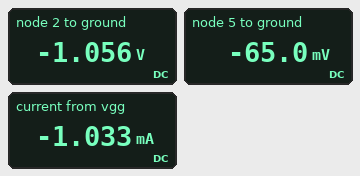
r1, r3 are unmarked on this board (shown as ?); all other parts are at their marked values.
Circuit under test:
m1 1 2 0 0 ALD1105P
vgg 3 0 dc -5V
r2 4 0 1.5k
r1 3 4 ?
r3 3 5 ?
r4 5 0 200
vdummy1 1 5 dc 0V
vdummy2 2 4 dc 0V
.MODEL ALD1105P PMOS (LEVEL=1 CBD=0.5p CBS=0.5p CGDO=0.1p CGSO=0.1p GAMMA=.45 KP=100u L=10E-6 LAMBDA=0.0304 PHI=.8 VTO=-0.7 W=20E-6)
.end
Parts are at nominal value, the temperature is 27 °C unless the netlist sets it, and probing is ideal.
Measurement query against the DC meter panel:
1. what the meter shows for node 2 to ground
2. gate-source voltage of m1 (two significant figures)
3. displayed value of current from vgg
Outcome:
-1.056 V
-1.1 V
-1.033 mA
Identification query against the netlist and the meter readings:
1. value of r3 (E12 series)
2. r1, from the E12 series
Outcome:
15 kΩ
5.6 kΩ
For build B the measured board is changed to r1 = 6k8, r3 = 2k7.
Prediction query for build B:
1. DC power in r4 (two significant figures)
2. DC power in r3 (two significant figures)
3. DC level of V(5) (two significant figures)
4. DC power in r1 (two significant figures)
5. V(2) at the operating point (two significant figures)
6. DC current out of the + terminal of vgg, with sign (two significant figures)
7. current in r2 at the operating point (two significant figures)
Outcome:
590 µW
8.0 mW
-340 mV
2.5 mW
-900 mV
-2.3 mA
600 µA
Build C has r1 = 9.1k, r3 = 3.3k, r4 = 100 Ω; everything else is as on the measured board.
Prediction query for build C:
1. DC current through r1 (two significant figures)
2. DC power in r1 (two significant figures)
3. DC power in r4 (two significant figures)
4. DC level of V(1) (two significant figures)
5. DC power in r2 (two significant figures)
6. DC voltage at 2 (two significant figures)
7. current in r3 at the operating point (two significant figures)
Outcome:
470 µA
2.0 mW
220 µW
-150 mV
330 µW
-710 mV
1.5 mA
